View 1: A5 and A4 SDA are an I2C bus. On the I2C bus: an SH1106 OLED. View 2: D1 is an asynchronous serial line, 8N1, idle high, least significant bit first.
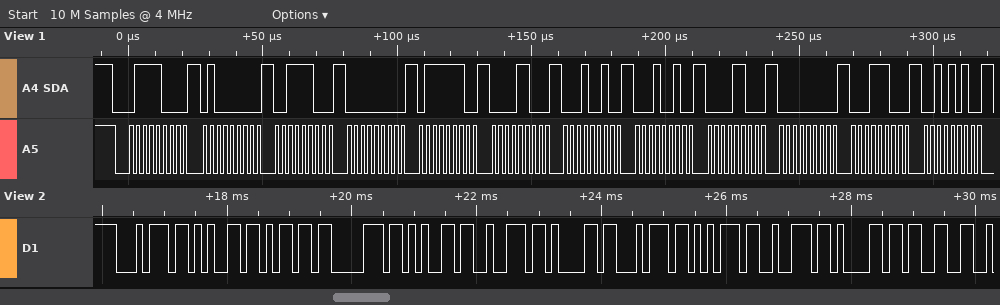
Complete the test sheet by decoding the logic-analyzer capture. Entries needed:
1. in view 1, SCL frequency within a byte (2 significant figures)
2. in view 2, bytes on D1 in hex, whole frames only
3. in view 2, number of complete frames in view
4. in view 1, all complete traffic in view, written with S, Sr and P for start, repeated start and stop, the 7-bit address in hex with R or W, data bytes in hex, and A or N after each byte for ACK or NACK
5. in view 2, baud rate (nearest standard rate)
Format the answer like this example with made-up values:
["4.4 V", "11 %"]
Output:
["400 kHz", "74 65 6D 70 65 72 61 74 75 72 61 33", "12", "S 3CW A 40 A 3C A 00 A 7E A 0C A 12 A 12 A 0C A 00 A 1C A 2A A", "9600 baud"]
